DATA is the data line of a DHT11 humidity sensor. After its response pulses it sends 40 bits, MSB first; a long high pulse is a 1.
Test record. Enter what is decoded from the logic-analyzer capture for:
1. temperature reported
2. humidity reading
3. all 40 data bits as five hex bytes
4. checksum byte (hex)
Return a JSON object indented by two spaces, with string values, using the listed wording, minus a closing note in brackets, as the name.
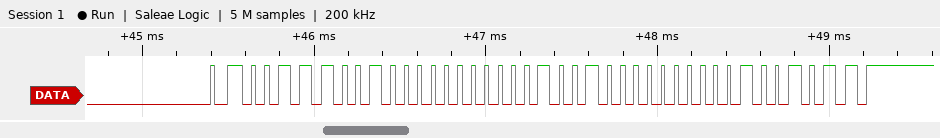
{
  "temperature reported": "18.0 °C",
  "humidity reading": "57 %",
  "all 40 data bits as five hex bytes": "39 00 12 00 4B",
  "checksum byte": "0x4B"
}
